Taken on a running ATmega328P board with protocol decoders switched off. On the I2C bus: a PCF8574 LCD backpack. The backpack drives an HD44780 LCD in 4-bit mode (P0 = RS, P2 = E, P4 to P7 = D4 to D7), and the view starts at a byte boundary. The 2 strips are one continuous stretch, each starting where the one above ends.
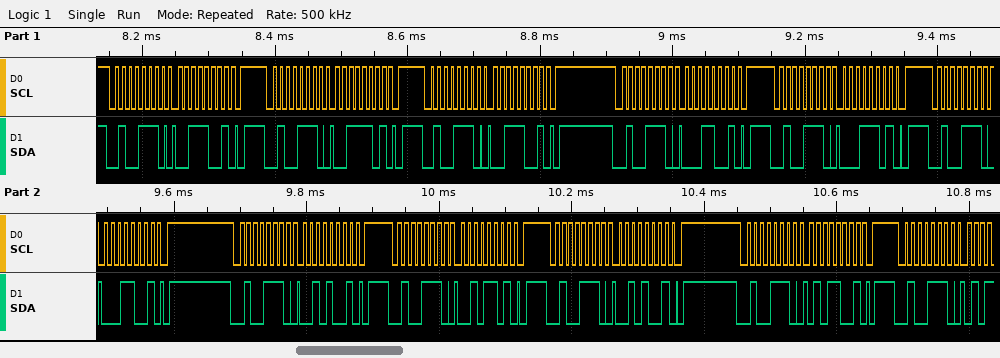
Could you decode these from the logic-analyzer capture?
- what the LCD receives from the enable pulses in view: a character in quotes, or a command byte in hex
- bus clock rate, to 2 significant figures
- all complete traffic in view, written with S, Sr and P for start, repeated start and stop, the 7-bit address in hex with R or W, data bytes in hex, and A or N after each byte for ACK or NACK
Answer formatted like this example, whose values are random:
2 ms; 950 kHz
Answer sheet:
'1'; 100 kHz; S 27W A 39 A P S 27W A 3D A P S 27W A 39 A P S 27W A 19 A P S 27W A 1D A P S 27W A 19 A P S 27W A 29 A P S 27W A 2D A P S 27W A 29 A P S 27W A 59 A P S 27W A
